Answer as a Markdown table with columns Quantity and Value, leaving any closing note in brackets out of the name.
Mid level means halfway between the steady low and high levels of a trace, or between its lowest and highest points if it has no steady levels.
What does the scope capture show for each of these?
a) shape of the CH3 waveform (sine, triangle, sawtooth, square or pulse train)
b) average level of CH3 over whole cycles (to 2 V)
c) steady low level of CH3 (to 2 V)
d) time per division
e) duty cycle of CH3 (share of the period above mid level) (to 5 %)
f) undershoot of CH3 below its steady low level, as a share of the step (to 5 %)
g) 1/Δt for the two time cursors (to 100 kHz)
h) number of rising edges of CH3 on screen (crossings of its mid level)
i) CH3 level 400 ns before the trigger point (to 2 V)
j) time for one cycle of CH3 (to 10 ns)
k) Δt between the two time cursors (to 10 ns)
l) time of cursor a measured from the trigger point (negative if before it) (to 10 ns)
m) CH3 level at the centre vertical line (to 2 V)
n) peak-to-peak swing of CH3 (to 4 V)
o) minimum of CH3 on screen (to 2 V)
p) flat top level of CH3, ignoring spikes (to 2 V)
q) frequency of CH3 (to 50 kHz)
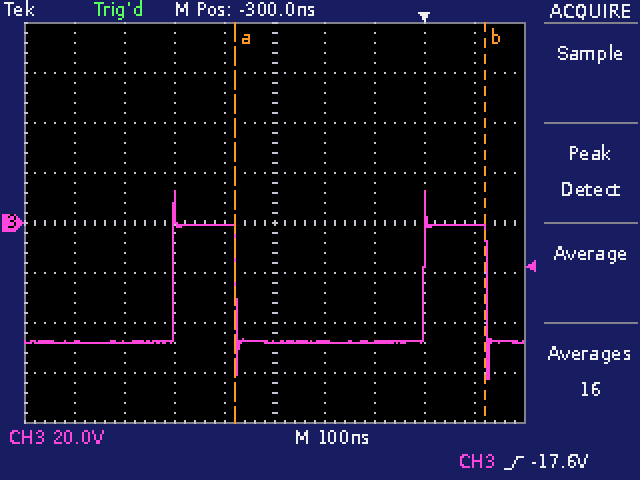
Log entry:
| Quantity | Value |
|---|---|
| shape of the CH3 waveform | pulse train |
| average level of CH3 over whole cycles | -36 V |
| steady low level of CH3 | -48 V |
| time per division | 100 ns |
| duty cycle of CH3 (share of the period above mid level) | 25 % |
| undershoot of CH3 below its steady low level, as a share of the step | 30 % |
| 1/Δt for the two time cursors | 2.0 MHz |
| number of rising edges of CH3 on screen | 2 |
| CH3 level 400 ns before the trigger point | 0 V |
| time for one cycle of CH3 | 500 ns |
| Δt between the two time cursors | 500 ns |
| time of cursor a measured from the trigger point (negative if before it) | -380 ns |
| CH3 level at the centre vertical line | -48 V |
| peak-to-peak swing of CH3 | 76 V |
| minimum of CH3 on screen | -62 V |
| flat top level of CH3, ignoring spikes | 0 V |
| frequency of CH3 | 2.00 MHz |
